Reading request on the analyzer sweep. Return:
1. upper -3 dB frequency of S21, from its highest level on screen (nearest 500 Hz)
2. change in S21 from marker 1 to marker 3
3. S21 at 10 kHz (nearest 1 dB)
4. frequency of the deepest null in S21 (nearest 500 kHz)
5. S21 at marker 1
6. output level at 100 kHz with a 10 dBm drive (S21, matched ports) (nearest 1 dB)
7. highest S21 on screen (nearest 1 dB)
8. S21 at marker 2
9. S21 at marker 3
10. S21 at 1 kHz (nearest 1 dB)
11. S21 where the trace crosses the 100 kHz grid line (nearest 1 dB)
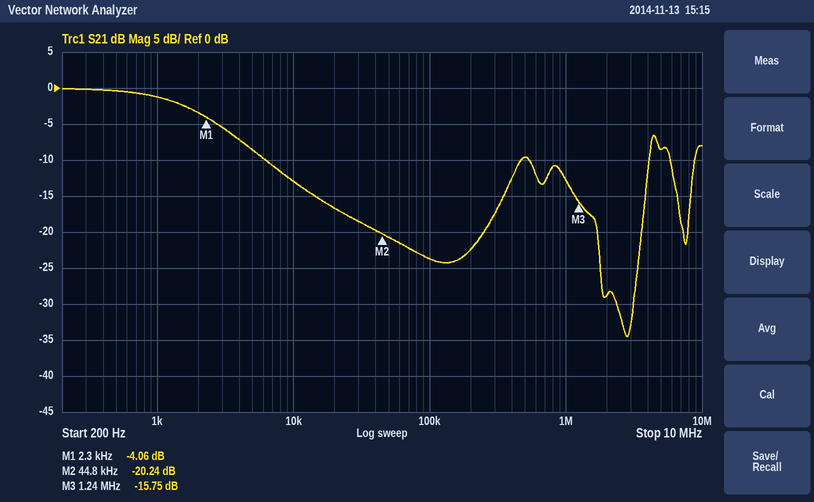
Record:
2.0 kHz
-11.69 dB
-13 dB
3.0 MHz
-4.06 dB
-14 dBm
0 dB
-20.24 dB
-15.75 dB
-1 dB
-24 dB
